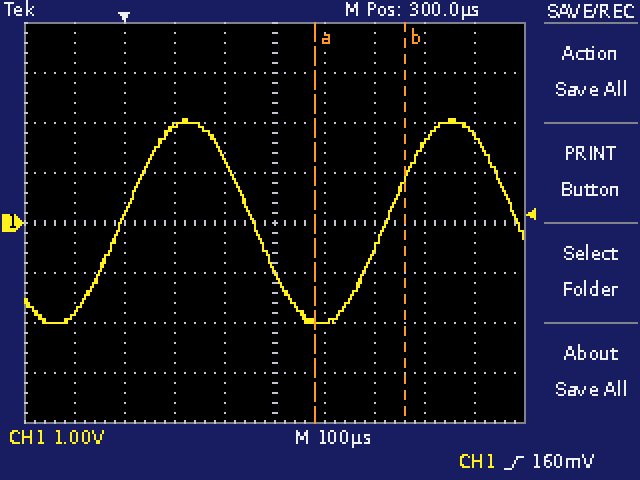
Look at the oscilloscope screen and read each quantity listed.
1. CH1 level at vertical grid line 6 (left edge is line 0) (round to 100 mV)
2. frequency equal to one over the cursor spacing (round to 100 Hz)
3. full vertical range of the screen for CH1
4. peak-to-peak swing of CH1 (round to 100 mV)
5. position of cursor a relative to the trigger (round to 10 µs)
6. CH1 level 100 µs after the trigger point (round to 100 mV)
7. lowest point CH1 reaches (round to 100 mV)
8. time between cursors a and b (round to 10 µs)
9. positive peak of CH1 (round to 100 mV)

-2.0 V
5.6 kHz
8 V
4.1 V
+380 µs
1.9 V
-2.0 V
180 µs
2.1 V
